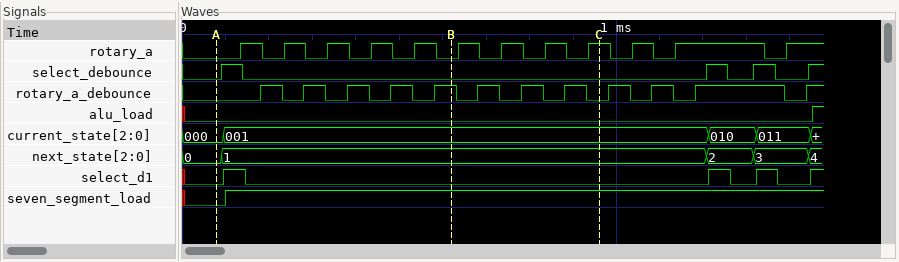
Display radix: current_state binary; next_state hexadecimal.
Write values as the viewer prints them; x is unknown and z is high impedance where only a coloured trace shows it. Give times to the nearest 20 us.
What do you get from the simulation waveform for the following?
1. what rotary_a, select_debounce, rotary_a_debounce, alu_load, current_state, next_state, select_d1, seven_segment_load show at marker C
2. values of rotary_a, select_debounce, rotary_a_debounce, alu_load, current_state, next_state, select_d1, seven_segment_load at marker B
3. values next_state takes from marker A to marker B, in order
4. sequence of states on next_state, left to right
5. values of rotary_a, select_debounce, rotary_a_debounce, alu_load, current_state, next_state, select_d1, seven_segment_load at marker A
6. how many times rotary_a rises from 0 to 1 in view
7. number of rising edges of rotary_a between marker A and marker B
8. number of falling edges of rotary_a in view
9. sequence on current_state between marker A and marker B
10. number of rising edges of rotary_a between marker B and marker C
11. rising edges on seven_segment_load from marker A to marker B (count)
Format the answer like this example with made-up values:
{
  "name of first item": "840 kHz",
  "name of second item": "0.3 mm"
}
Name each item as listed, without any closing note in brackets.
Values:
{
  "what rotary_a, select_debounce, rotary_a_debounce, alu_load, current_state, next_state, select_d1, seven_segment_load show at marker C": "rotary_a=1, select_debounce=0, rotary_a_debounce=0, alu_load=0, current_state=001, next_state=1, select_d1=0, seven_segment_load=1",
  "values of rotary_a, select_debounce, rotary_a_debounce, alu_load, current_state, next_state, select_d1, seven_segment_load at marker B": "rotary_a=0, select_debounce=0, rotary_a_debounce=1, alu_load=0, current_state=001, next_state=1, select_d1=0, seven_segment_load=1",
  "values next_state takes from marker A to marker B, in order": "0, 1",
  "sequence of states on next_state, left to right": "0, 1, 2, 3, 4",
  "values of rotary_a, select_debounce, rotary_a_debounce, alu_load, current_state, next_state, select_d1, seven_segment_load at marker A": "rotary_a=0, select_debounce=0, rotary_a_debounce=0, alu_load=0, current_state=000, next_state=0, select_d1=0, seven_segment_load=0",
  "how many times rotary_a rises from 0 to 1 in view": "12",
  "number of rising edges of rotary_a between marker A and marker B": "5",
  "number of falling edges of rotary_a in view": "11",
  "sequence on current_state between marker A and marker B": "000, 001",
  "number of rising edges of rotary_a between marker B and marker C": "4",
  "rising edges on seven_segment_load from marker A to marker B": "1"
}
